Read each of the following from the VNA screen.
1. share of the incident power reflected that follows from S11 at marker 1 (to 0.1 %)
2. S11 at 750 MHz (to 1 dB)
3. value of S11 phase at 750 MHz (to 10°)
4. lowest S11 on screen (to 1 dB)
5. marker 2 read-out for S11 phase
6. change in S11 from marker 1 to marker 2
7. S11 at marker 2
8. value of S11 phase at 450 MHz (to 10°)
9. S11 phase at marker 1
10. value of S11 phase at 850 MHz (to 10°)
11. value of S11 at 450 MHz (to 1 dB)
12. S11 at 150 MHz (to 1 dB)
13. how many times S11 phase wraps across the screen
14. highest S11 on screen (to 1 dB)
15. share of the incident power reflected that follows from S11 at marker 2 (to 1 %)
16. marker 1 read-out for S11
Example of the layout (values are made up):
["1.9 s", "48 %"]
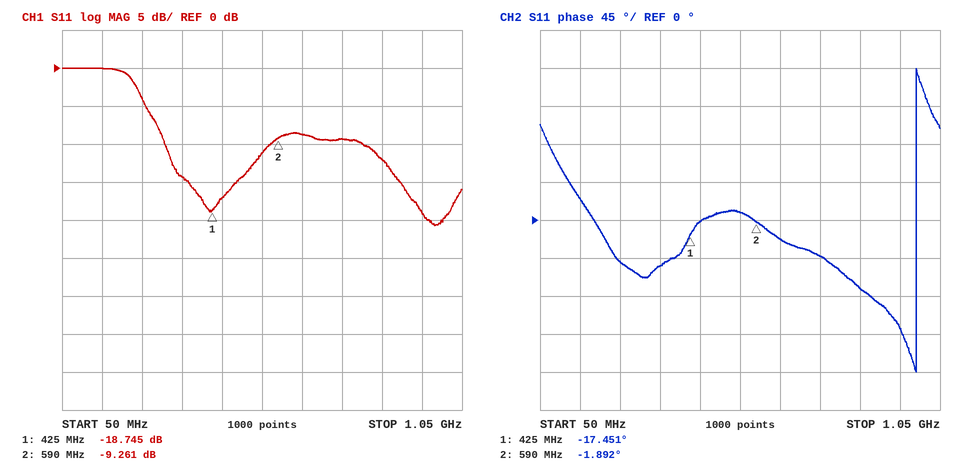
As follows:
["1.3 %", "-9 dB", "-40°", "-21 dB", "-1.892°", "9.484 dB", "-9.261 dB", "0°", "-17.451°", "-80°", "-17 dB", "0 dB", "1", "0 dB", "12 %", "-18.745 dB"]
